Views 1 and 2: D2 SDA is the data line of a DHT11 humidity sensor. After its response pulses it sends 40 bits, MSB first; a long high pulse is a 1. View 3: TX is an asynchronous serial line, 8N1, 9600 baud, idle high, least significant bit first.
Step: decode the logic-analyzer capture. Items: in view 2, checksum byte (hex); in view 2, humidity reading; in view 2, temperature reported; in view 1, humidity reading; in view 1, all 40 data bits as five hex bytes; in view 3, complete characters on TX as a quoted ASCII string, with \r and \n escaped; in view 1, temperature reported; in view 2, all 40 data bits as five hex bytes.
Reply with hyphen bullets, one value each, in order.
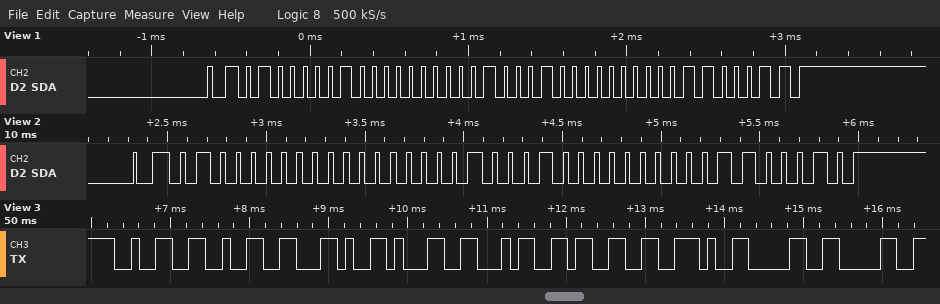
- 0x62
- 64 %
- 34.0 °C
- 65 %
- 41 00 22 00 63
- "22,143.00"
- 34.0 °C
- 40 00 22 00 62
